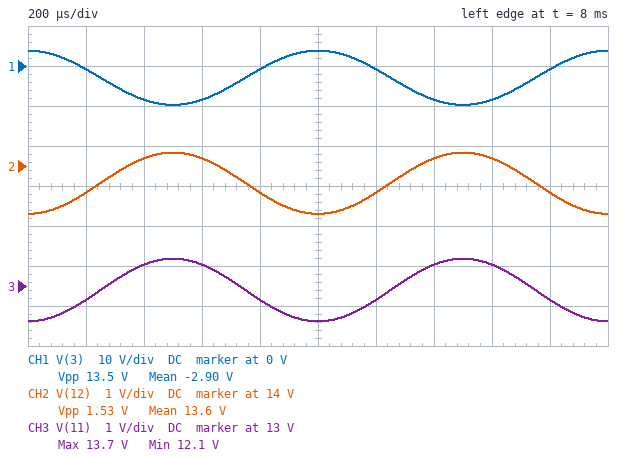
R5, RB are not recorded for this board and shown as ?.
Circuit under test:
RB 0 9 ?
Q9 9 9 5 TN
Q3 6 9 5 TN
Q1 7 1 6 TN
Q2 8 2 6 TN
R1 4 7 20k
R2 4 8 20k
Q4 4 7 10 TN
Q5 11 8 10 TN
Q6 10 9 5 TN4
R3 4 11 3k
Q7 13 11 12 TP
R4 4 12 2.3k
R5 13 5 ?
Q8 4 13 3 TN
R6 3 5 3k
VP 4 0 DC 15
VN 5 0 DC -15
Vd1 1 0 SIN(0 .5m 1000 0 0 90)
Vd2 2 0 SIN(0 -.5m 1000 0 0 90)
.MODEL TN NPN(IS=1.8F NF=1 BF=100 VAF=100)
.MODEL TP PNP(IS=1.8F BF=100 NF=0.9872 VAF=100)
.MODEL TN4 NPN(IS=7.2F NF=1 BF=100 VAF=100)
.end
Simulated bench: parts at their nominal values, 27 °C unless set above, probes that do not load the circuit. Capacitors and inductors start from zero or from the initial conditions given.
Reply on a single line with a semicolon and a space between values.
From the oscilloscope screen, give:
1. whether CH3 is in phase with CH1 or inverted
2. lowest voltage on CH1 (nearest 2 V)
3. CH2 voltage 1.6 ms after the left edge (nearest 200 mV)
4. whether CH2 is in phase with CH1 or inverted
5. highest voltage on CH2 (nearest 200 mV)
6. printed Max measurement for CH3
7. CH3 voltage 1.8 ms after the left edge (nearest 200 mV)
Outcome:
inverted; -10 V; 14.2 V; inverted; 14.4 V; 13.7 V; 12.6 V
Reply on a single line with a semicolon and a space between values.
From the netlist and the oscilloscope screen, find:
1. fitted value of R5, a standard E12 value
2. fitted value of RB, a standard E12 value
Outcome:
22 kΩ; 47 kΩ
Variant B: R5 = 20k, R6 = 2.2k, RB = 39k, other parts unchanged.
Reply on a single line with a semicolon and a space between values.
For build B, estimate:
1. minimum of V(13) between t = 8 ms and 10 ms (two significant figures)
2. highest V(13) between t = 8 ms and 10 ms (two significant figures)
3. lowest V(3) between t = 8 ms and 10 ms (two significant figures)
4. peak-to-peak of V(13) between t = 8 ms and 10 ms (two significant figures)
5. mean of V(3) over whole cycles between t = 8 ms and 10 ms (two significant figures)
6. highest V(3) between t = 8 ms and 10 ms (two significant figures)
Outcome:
-7.9 V; 7.2 V; -8.6 V; 15 V; -1.1 V; 6.4 V
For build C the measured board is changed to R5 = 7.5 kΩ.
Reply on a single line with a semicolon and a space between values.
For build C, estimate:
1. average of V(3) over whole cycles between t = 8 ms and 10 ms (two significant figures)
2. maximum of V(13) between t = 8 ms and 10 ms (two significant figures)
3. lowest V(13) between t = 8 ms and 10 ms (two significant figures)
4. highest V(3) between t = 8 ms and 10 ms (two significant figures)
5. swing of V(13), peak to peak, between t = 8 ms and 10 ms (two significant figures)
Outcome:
-11 V; -8.0 V; -13 V; -8.7 V; 4.9 V
